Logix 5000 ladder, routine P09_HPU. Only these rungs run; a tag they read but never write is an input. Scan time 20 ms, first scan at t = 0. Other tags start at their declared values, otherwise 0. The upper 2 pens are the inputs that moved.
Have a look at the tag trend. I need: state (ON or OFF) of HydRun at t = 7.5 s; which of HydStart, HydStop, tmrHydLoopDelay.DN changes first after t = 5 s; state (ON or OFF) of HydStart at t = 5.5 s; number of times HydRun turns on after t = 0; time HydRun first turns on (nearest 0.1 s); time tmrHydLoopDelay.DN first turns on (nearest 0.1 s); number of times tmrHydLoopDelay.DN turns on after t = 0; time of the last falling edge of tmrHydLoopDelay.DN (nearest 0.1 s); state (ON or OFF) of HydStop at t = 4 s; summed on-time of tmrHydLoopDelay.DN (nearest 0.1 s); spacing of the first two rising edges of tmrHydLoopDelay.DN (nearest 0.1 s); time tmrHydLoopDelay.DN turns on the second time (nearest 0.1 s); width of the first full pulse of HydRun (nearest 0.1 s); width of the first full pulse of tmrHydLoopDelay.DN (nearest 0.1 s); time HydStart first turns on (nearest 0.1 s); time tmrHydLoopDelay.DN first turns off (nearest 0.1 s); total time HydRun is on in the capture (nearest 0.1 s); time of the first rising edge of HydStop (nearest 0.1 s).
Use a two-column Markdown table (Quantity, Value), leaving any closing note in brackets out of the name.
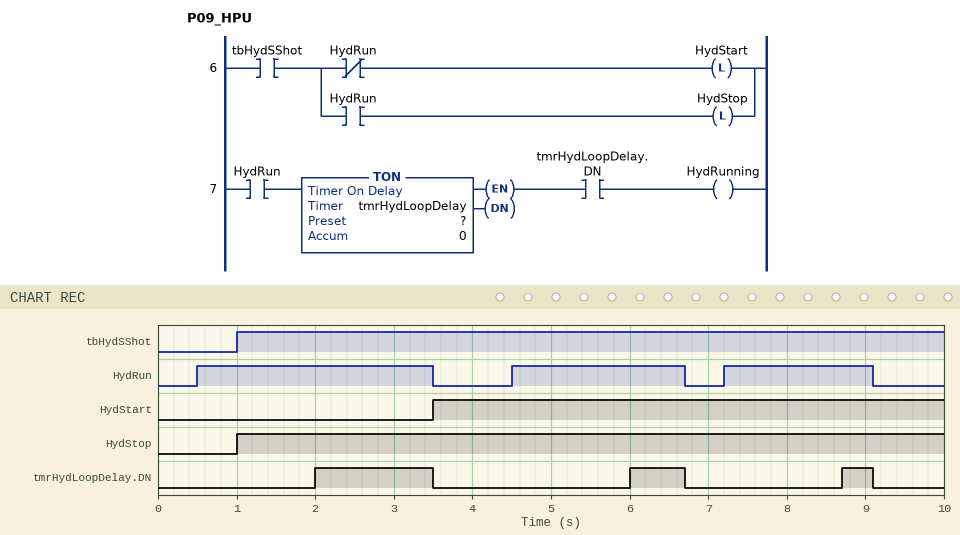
| Quantity | Value |
|---|---|
| state (ON or OFF) of HydRun at t = 7.5 s | ON |
| which of HydStart, HydStop, tmrHydLoopDelay.DN changes first after t = 5 s | tmrHydLoopDelay.DN |
| state (ON or OFF) of HydStart at t = 5.5 s | ON |
| number of times HydRun turns on after t = 0 | 3 |
| time HydRun first turns on | 0.5 s |
| time tmrHydLoopDelay.DN first turns on | 2.0 s |
| number of times tmrHydLoopDelay.DN turns on after t = 0 | 3 |
| time of the last falling edge of tmrHydLoopDelay.DN | 9.1 s |
| state (ON or OFF) of HydStop at t = 4 s | ON |
| summed on-time of tmrHydLoopDelay.DN | 2.6 s |
| spacing of the first two rising edges of tmrHydLoopDelay.DN | 4.0 s |
| time tmrHydLoopDelay.DN turns on the second time | 6.0 s |
| width of the first full pulse of HydRun | 3.0 s |
| width of the first full pulse of tmrHydLoopDelay.DN | 1.5 s |
| time HydStart first turns on | 3.5 s |
| time tmrHydLoopDelay.DN first turns off | 3.5 s |
| total time HydRun is on in the capture | 7.1 s |
| time of the first rising edge of HydStop | 1.0 s |
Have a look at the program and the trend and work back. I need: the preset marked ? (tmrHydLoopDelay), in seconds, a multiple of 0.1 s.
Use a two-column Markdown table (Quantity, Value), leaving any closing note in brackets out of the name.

| Quantity | Value |
|---|---|
| the preset marked ? (tmrHydLoopDelay), in seconds, a multiple of 0.1 s | 1.5 s |
